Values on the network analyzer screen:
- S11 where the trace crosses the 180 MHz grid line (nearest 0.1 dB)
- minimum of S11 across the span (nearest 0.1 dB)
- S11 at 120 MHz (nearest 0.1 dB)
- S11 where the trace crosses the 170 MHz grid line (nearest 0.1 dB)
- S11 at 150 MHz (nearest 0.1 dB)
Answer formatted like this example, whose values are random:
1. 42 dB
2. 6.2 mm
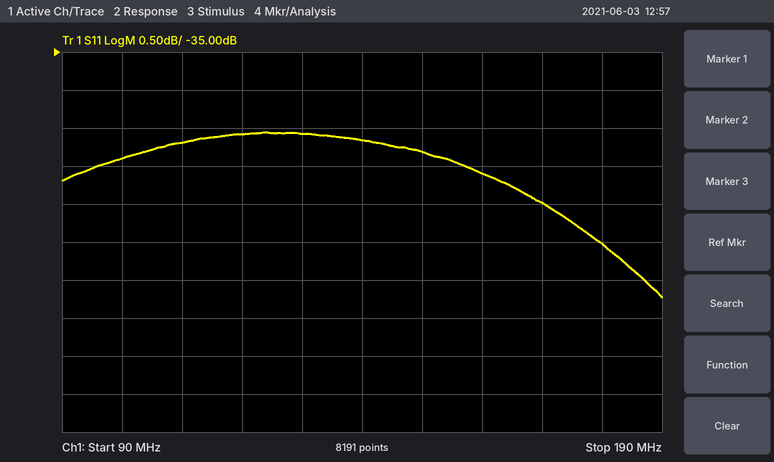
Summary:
1. -37.5 dB
2. -38.2 dB
3. -36.1 dB
4. -37.0 dB
5. -36.3 dB
